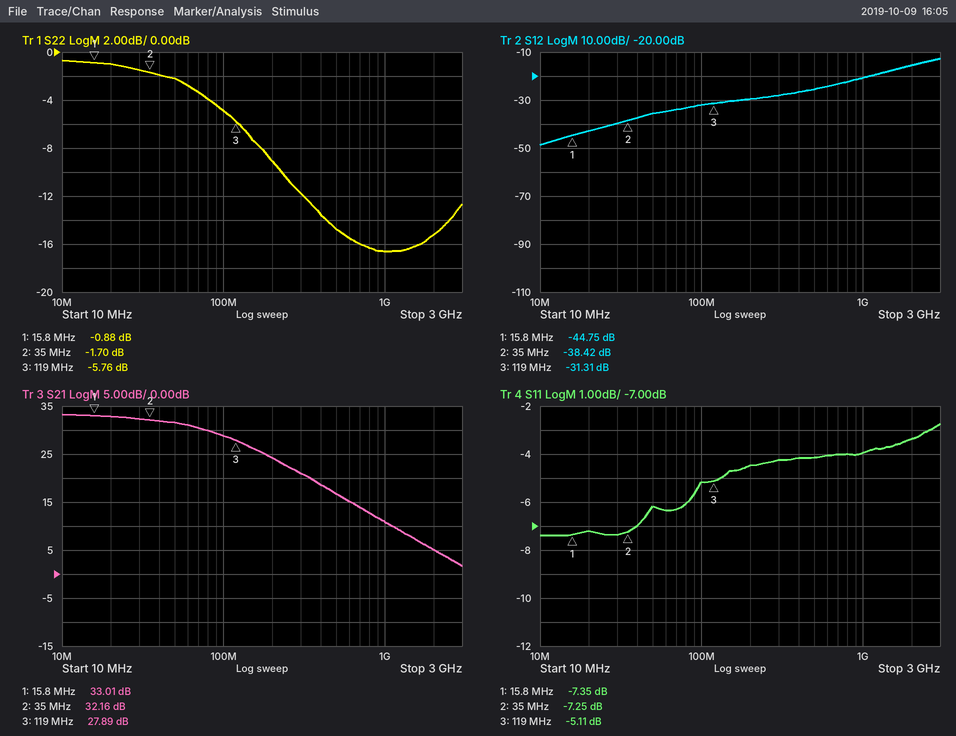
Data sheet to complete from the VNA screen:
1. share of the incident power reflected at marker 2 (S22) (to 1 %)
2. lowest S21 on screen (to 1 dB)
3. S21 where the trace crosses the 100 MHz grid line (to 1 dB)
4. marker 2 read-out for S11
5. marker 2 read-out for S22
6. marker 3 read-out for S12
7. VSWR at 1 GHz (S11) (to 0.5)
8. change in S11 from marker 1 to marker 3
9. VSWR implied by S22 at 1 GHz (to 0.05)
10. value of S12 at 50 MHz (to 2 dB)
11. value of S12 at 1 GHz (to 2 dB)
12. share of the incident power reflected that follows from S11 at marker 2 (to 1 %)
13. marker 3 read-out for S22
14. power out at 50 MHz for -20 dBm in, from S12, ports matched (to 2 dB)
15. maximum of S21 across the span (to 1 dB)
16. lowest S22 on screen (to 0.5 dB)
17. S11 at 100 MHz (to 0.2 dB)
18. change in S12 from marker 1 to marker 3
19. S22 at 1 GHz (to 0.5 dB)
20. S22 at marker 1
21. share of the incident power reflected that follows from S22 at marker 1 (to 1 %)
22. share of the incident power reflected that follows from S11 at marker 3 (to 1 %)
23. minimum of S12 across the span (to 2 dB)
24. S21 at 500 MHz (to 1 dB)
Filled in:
68 %
2 dB
29 dB
-7.25 dB
-1.70 dB
-31.31 dB
4.5
2.24 dB
1.35
-36 dB
-20 dB
19 %
-5.76 dB
-56 dBm
33 dB
-16.5 dB
-5.2 dB
13.44 dB
-16.5 dB
-0.88 dB
82 %
31 %
-48 dB
17 dB
